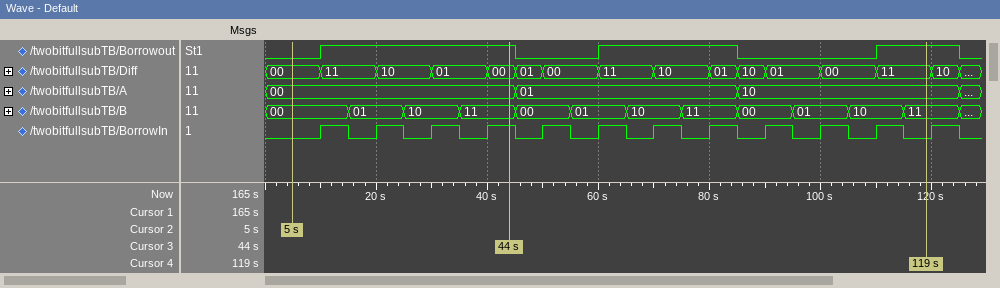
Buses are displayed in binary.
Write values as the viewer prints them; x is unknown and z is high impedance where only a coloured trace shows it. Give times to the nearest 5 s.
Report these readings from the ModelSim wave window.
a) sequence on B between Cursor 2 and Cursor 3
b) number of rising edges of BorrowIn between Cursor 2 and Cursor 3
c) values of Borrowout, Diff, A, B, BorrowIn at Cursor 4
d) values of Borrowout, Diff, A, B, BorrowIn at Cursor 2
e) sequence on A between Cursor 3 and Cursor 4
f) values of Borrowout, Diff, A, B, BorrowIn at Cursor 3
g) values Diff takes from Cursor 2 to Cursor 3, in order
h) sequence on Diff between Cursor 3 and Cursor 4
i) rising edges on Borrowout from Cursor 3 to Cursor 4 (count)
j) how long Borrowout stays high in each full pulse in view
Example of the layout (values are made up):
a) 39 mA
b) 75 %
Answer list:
a) 00, 01, 10, 11
b) 4
c) Borrowout=1, Diff=11, A=10, B=11, BorrowIn=0
d) Borrowout=0, Diff=00, A=00, B=00, BorrowIn=0
e) 00, 01, 10
f) Borrowout=1, Diff=00, A=00, B=11, BorrowIn=1
g) 00, 11, 10, 01, 00
h) 00, 01, 00, 11, 10, 01, 10, 01, 00, 11
i) 2
j) 35 s, 25 s, 15 s
